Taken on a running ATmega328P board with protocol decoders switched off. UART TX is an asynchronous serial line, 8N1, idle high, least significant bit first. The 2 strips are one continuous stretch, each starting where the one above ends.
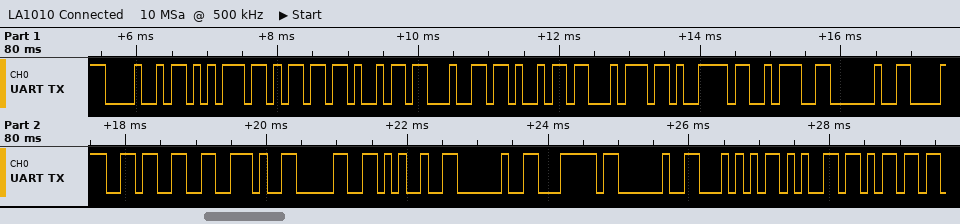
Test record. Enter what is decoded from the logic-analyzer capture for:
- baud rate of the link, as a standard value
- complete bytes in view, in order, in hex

9600 baud
0x48 0x75 0x6D 0x69 0x64 0x69 0x74 0x79 0x3A 0x20 0x38 0x33 0x2E 0x30 0x25 0x20 0x7C 0x20 0x54 0x65 0x6D
